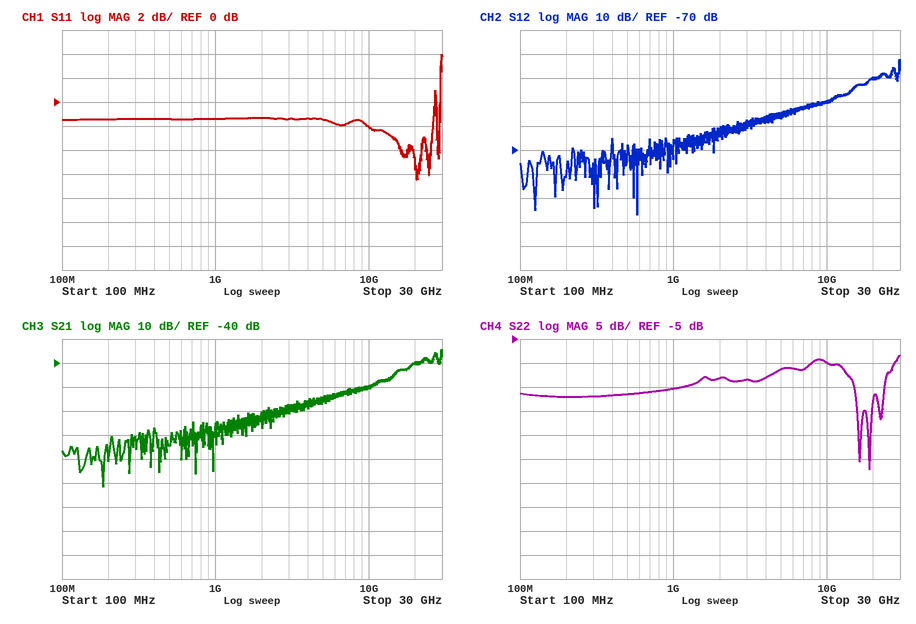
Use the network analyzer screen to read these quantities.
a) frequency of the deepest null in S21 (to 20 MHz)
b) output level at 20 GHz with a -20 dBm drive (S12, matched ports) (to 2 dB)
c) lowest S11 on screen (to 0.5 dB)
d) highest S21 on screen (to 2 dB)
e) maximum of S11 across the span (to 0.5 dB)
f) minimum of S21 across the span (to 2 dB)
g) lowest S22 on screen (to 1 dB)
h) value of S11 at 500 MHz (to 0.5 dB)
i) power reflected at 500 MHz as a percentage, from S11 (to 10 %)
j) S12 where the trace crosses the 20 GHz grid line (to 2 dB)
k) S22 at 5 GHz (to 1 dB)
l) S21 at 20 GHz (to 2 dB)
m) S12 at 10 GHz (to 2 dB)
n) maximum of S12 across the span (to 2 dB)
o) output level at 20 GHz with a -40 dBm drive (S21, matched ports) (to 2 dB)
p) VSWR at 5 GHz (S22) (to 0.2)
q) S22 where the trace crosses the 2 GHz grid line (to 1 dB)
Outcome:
180 MHz
-60 dBm
-6.5 dB
-34 dB
4.0 dB
-92 dB
-32 dB
-1.5 dB
70 %
-40 dB
-11 dB
-40 dB
-50 dB
-32 dB
-80 dBm
1.8
-13 dB
